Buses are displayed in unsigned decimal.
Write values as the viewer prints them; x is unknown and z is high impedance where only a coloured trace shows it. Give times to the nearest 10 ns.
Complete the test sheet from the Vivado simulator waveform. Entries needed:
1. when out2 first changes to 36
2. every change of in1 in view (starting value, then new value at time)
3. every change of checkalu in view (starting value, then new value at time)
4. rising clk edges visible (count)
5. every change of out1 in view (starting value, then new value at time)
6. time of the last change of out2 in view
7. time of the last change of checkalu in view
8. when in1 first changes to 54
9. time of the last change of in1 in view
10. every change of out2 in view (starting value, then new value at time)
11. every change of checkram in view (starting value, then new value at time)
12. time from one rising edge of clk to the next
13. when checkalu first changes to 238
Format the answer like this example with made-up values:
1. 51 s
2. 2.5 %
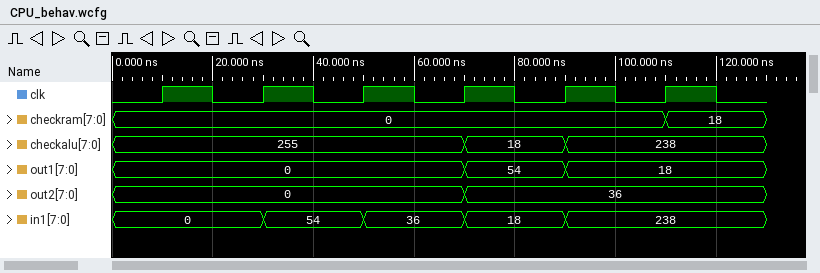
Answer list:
1. 70 ns
2. 0, 54 at 30 ns, 36 at 50 ns, 18 at 70 ns, 238 at 90 ns
3. 255, 18 at 70 ns, 238 at 90 ns
4. 6
5. 0, 54 at 70 ns, 18 at 90 ns
6. 70 ns
7. 90 ns
8. 30 ns
9. 90 ns
10. 0, 36 at 70 ns
11. 0, 18 at 110 ns
12. 20 ns
13. 90 ns
